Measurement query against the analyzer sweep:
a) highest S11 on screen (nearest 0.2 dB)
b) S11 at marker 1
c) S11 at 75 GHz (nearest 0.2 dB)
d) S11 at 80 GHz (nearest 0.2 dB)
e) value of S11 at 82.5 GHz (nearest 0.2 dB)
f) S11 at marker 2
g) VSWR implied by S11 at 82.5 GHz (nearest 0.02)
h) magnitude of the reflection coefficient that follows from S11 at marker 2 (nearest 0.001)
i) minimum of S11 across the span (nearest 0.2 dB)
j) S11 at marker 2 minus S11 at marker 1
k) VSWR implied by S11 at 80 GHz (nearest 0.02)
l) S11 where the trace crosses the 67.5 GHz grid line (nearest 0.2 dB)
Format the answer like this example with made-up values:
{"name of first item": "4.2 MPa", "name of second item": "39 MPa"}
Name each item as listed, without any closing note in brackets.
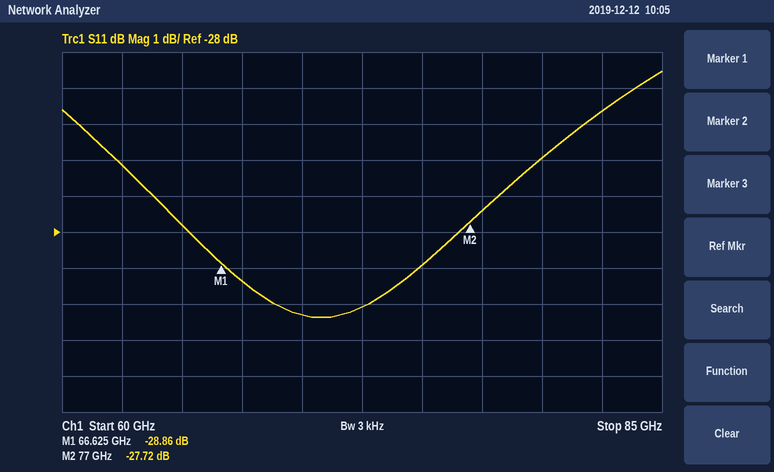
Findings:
{"highest S11 on screen": "-23.6 dB", "S11 at marker 1": "-28.86 dB", "S11 at 75 GHz": "-29.0 dB", "S11 at 80 GHz": "-26.0 dB", "value of S11 at 82.5 GHz": "-24.6 dB", "S11 at marker 2": "-27.72 dB", "VSWR implied by S11 at 82.5 GHz": "1.12", "magnitude of the reflection coefficient that follows from S11 at marker 2": "0.041", "minimum of S11 across the span": "-30.4 dB", "S11 at marker 2 minus S11 at marker 1": "1.14 dB", "VSWR implied by S11 at 80 GHz": "1.10", "S11 where the trace crosses the 67.5 GHz grid line": "-29.4 dB"}
